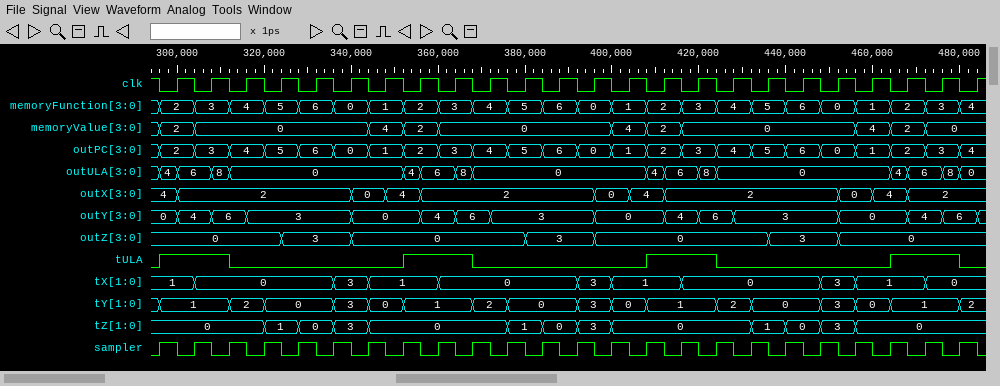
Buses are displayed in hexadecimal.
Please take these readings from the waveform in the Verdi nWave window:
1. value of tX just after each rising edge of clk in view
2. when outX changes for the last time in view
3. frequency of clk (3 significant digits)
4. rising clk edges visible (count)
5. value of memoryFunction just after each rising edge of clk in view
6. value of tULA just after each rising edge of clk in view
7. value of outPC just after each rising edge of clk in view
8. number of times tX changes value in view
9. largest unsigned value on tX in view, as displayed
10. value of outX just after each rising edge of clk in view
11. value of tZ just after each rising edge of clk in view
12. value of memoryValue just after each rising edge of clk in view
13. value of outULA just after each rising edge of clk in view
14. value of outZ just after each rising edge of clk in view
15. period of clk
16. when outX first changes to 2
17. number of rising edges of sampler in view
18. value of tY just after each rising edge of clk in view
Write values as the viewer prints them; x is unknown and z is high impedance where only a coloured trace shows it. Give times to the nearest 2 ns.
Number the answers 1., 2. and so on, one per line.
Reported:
1. 1, 0, 0, 0, 0, 3, 1, 1, 0, 0, 0, 0, 3, 1, 1, 0, 0, 0, 0, 3, 1, 1, 0, 0
2. 468 ns
3. 125 MHz
4. 24
5. 2, 3, 4, 5, 6, 0, 1, 2, 3, 4, 5, 6, 0, 1, 2, 3, 4, 5, 6, 0, 1, 2, 3, 4
6. 1 1 0 0 0 0 0 1 1 0 0 0 0 0 1 1 0 0 0 0 0 1 1 0
7. 2, 3, 4, 5, 6, 0, 1, 2, 3, 4, 5, 6, 0, 1, 2, 3, 4, 5, 6, 0, 1, 2, 3, 4
8. 10
9. 3
10. 2, 2, 2, 2, 2, 0, 4, 2, 2, 2, 2, 2, 0, 4, 2, 2, 2, 2, 2, 0, 4, 2, 2, 2
11. 0, 0, 0, 1, 0, 3, 0, 0, 0, 0, 1, 0, 3, 0, 0, 0, 0, 1, 0, 3, 0, 0, 0, 0
12. 2, 0, 0, 0, 0, 0, 4, 2, 0, 0, 0, 0, 0, 4, 2, 0, 0, 0, 0, 0, 4, 2, 0, 0
13. 6, 8, 0, 0, 0, 0, 0, 6, 8, 0, 0, 0, 0, 0, 6, 8, 0, 0, 0, 0, 0, 6, 8, 0
14. 0, 0, 0, 3, 3, 0, 0, 0, 0, 0, 3, 3, 0, 0, 0, 0, 0, 3, 3, 0, 0, 0, 0, 0
15. 8 ns
16. 300 ns
17. 24
18. 1, 1, 2, 0, 0, 3, 0, 1, 1, 2, 0, 0, 3, 0, 1, 1, 2, 0, 0, 3, 0, 1, 1, 2
